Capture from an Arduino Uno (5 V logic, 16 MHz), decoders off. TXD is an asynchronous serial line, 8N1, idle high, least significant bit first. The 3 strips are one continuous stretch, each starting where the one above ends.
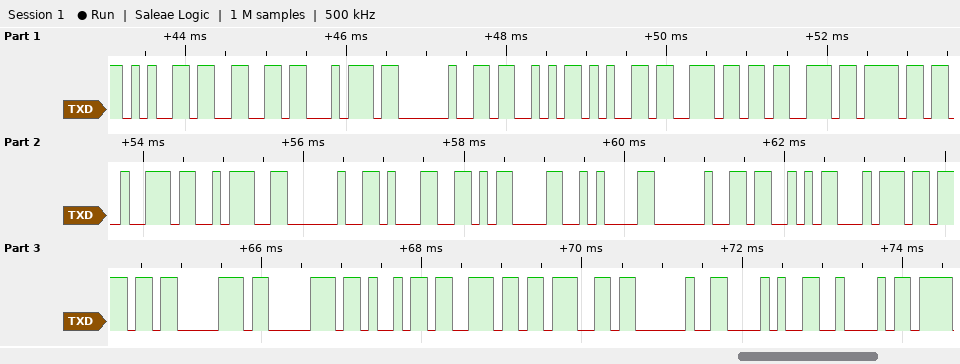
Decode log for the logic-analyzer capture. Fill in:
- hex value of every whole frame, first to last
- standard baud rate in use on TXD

65 66 74 20 53 65 6E 73 6F 72 3A 20 31 0D 0A 20 53 74 6F 70 70 69 6E 67 20 28 42
9600 baud
